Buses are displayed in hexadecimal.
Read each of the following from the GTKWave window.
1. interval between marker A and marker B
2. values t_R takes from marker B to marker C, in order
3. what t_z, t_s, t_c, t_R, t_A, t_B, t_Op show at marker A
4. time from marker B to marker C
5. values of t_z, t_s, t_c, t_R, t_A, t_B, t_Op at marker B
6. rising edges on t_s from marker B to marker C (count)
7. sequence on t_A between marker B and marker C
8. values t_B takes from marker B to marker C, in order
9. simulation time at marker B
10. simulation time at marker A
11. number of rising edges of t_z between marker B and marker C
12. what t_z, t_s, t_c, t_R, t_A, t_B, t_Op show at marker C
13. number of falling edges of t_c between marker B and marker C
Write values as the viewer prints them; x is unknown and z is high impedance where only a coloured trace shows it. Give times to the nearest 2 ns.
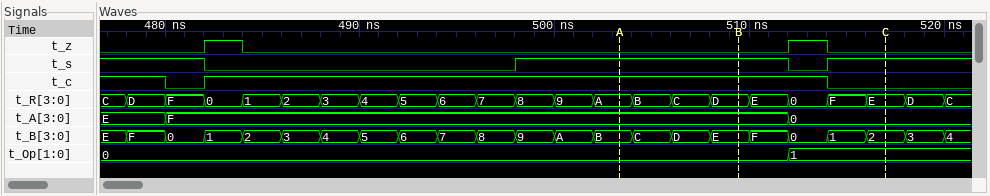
6 ns
D, E, 0, F, E
t_z=0, t_s=1, t_c=1, t_R=A, t_A=F, t_B=B, t_Op=0
8 ns
t_z=0, t_s=1, t_c=1, t_R=D, t_A=F, t_B=E, t_Op=0
1
F, 0
E, F, 0, 1, 2
510 ns
504 ns
1
t_z=0, t_s=1, t_c=0, t_R=E, t_A=0, t_B=2, t_Op=1
1
